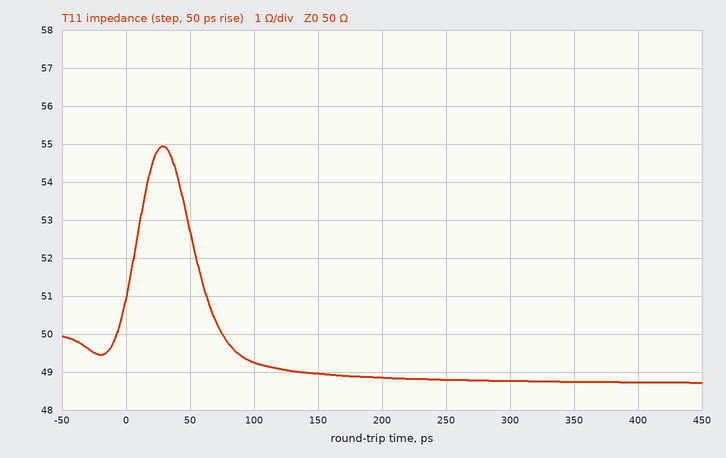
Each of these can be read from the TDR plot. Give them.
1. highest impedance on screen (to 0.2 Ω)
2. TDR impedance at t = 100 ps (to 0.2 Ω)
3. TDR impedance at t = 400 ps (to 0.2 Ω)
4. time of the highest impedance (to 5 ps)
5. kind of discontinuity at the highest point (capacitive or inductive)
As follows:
55.0 Ω
49.2 Ω
48.8 Ω
30 ps
inductive
